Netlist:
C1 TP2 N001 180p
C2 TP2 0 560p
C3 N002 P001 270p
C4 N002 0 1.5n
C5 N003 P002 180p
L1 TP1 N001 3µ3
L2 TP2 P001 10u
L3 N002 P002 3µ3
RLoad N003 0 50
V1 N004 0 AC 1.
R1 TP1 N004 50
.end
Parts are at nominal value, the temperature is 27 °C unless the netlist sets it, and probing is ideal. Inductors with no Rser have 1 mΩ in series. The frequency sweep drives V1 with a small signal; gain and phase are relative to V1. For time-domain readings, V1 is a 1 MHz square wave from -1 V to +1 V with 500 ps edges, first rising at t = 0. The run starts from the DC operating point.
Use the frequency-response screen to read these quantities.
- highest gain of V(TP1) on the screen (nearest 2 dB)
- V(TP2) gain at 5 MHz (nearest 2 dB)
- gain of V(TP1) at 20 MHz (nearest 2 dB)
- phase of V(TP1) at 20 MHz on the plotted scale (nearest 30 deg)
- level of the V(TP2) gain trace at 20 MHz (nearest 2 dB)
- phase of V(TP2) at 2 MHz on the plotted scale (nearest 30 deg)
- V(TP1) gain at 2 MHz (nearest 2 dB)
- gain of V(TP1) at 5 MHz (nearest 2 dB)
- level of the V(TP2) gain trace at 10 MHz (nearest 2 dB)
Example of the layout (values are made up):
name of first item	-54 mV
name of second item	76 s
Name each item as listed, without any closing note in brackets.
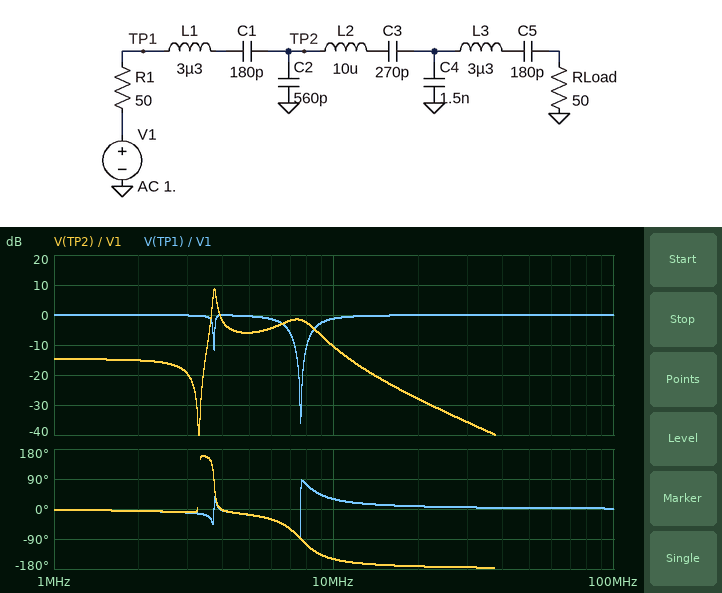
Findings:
highest gain of V(TP1) on the screen	0 dB
V(TP2) gain at 5 MHz	-6 dB
gain of V(TP1) at 20 MHz	0 dB
phase of V(TP1) at 20 MHz on the plotted scale	0 deg
level of the V(TP2) gain trace at 20 MHz	-28 dB
phase of V(TP2) at 2 MHz on the plotted scale	0 deg
V(TP1) gain at 2 MHz	0 dB
gain of V(TP1) at 5 MHz	0 dB
level of the V(TP2) gain trace at 10 MHz	-10 dB
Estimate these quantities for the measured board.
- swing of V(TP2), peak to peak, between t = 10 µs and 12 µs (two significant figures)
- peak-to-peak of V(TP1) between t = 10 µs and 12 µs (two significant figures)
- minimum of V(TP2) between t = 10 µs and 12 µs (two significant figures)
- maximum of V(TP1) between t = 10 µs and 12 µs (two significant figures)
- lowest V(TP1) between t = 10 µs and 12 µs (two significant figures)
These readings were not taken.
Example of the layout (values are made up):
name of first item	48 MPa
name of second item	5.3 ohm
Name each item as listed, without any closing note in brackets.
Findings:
swing of V(TP2), peak to peak, between t = 10 µs and 12 µs	960 mV
peak-to-peak of V(TP1) between t = 10 µs and 12 µs	2.6 V
minimum of V(TP2) between t = 10 µs and 12 µs	-300 mV
maximum of V(TP1) between t = 10 µs and 12 µs	1.3 V
lowest V(TP1) between t = 10 µs and 12 µs	-1.3 V
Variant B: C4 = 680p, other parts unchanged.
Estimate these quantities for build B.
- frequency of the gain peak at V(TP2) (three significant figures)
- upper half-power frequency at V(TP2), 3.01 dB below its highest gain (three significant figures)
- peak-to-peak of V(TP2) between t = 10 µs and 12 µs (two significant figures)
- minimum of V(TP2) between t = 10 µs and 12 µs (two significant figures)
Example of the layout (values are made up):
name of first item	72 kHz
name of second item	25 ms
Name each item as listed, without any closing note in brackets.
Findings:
frequency of the gain peak at V(TP2)	3.91 MHz
upper half-power frequency at V(TP2), 3.01 dB below its highest gain	4.00 MHz
peak-to-peak of V(TP2) between t = 10 µs and 12 µs	1.0 V
minimum of V(TP2) between t = 10 µs and 12 µs	-310 mV
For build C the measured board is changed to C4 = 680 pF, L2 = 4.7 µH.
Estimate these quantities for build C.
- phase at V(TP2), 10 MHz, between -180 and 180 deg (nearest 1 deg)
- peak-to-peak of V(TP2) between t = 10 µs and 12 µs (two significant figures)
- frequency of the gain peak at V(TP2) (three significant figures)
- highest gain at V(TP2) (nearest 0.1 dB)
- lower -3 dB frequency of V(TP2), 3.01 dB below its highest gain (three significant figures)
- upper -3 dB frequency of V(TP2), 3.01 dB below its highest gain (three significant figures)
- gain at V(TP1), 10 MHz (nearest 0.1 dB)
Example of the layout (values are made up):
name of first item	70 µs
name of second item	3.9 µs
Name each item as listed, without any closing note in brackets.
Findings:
phase at V(TP2), 10 MHz, between -180 and 180 deg	-150 deg
peak-to-peak of V(TP2) between t = 10 µs and 12 µs	830 mV
frequency of the gain peak at V(TP2)	7.67 MHz
highest gain at V(TP2)	-0.1 dB
lower -3 dB frequency of V(TP2), 3.01 dB below its highest gain	5.50 MHz
upper -3 dB frequency of V(TP2), 3.01 dB below its highest gain	8.60 MHz
gain at V(TP1), 10 MHz	-1.3 dB
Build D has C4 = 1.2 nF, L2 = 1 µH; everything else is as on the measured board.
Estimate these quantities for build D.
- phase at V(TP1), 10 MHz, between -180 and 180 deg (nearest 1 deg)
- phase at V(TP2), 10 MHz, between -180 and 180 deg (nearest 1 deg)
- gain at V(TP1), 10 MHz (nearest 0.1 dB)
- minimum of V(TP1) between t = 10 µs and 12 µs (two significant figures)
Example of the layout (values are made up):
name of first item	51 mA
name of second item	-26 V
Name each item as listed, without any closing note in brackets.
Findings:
phase at V(TP1), 10 MHz, between -180 and 180 deg	24 deg
phase at V(TP2), 10 MHz, between -180 and 180 deg	-153 deg
gain at V(TP1), 10 MHz	-0.8 dB
minimum of V(TP1) between t = 10 µs and 12 µs	-1.3 V
